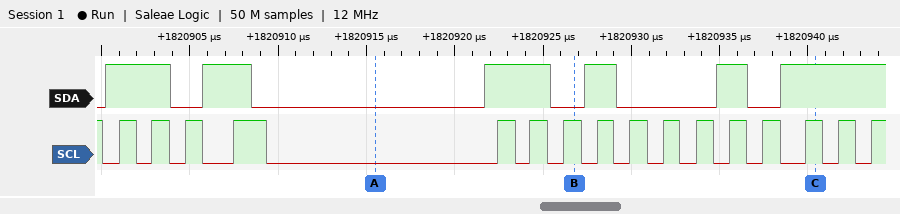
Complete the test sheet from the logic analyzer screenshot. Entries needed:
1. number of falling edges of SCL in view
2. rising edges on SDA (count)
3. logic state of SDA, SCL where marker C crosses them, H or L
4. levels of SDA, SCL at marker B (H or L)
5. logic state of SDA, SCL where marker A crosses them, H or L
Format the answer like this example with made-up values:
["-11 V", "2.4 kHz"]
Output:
["16", "6", "SDA=H, SCL=H", "SDA=L, SCL=H", "SDA=L, SCL=L"]
